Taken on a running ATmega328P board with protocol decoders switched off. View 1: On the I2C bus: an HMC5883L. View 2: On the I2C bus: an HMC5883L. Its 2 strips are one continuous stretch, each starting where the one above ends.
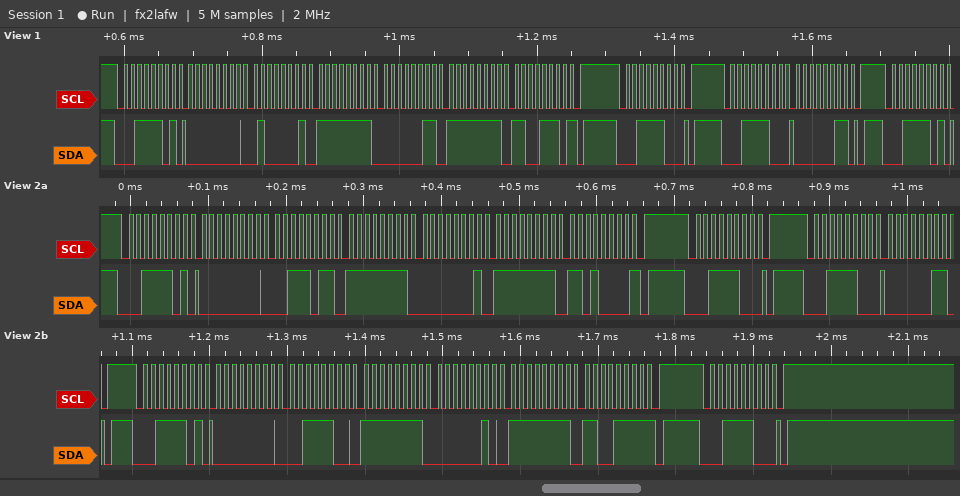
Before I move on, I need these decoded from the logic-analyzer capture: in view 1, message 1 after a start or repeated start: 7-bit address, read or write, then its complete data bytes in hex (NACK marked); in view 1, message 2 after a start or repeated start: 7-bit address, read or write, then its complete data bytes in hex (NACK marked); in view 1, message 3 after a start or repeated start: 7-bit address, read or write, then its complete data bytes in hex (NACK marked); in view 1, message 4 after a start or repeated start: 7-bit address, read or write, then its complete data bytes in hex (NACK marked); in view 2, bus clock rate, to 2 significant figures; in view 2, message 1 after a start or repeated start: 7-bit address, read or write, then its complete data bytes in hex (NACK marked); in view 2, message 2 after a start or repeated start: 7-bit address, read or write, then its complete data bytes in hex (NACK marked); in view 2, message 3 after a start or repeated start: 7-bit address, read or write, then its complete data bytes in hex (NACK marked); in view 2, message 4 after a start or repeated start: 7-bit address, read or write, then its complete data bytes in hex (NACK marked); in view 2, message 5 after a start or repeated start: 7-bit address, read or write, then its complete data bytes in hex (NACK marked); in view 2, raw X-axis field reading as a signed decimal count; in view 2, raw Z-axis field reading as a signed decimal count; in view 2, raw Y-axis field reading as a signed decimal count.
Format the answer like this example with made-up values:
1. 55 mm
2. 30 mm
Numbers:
1. 0x1E read: 00 41 FF 03 FF CE NACK
2. 0x1E write
3. 0x1E write: 03
4. 0x1E read
5. 100 kHz
6. 0x1E read: 00 3B FF 01 FF D0 NACK
7. 0x1E write
8. 0x1E write: 03
9. 0x1E read: 00 3C FF 02 FF CF NACK
10. 0x1E write
11. 60
12. -254
13. -49
